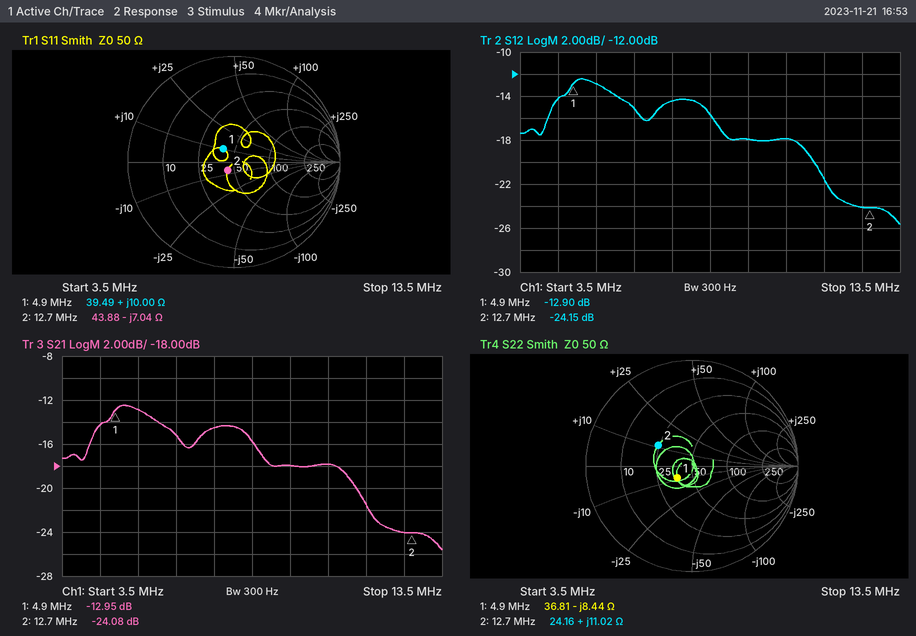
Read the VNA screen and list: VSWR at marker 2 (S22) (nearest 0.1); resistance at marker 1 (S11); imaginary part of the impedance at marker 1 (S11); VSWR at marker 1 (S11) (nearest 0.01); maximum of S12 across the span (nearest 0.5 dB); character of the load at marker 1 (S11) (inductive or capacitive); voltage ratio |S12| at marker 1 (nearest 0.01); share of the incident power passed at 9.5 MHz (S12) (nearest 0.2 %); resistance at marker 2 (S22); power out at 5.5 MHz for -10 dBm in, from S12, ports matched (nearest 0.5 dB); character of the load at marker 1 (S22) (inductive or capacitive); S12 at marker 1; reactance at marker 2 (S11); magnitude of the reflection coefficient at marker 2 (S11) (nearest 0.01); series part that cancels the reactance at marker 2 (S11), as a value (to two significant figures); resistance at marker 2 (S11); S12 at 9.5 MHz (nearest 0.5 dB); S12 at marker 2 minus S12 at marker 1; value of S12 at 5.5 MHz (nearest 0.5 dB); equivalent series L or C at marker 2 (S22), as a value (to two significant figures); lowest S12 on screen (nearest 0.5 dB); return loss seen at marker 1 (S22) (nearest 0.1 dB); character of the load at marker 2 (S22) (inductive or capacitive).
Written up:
2.2
39.49 Ω
+10.00 Ω
1.38
-12.5 dB
inductive
0.23
1.6 %
24.16 Ω
-23.0 dBm
capacitive
-12.90 dB
-7.04 Ω
0.10
88 nH
43.88 Ω
-18.0 dB
-11.25 dB
-13.0 dB
140 nH
-25.5 dB
14.9 dB
inductive
